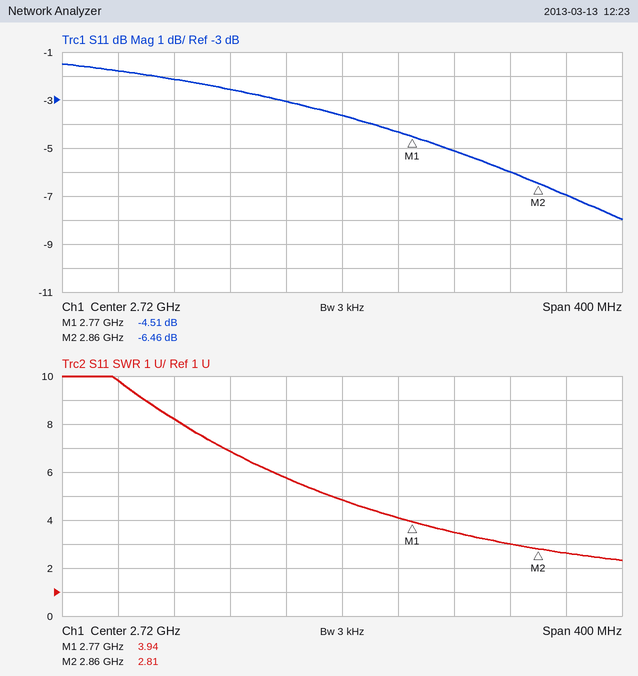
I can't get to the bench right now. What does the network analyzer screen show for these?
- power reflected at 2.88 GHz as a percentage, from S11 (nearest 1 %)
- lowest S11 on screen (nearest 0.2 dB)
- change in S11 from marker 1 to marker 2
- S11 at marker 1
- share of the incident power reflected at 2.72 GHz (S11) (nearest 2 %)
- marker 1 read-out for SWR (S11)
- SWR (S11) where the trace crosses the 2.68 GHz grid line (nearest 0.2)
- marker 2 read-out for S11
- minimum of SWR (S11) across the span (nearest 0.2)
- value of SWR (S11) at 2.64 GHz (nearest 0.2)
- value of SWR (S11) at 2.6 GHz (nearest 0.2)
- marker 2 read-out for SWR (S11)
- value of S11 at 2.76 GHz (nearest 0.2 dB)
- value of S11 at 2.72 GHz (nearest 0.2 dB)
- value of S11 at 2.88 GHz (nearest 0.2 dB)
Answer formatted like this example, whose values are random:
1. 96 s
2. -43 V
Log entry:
1. 20 %
2. -8.0 dB
3. -1.95 dB
4. -4.51 dB
5. 44 %
6. 3.94
7. 5.8
8. -6.46 dB
9. 2.4
10. 6.8
11. 8.2
12. 2.81
13. -4.4 dB
14. -3.6 dB
15. -7.0 dB
